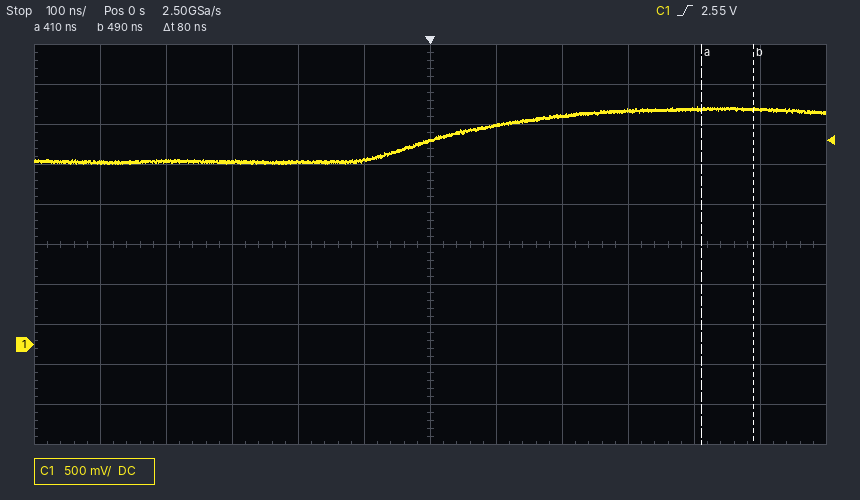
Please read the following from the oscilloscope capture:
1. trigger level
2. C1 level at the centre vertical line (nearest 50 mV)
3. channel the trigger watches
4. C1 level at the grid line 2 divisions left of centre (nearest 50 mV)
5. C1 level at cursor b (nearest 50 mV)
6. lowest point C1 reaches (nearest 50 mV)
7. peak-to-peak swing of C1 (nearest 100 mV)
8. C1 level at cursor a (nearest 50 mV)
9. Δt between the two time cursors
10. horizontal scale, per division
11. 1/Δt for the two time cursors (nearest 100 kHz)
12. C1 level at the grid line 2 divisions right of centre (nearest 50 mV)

2.55 V
2.55 V
C1
2.30 V
2.95 V
2.25 V
700 mV
2.95 V
80 ns
100 ns
12.5 MHz
2.85 V
